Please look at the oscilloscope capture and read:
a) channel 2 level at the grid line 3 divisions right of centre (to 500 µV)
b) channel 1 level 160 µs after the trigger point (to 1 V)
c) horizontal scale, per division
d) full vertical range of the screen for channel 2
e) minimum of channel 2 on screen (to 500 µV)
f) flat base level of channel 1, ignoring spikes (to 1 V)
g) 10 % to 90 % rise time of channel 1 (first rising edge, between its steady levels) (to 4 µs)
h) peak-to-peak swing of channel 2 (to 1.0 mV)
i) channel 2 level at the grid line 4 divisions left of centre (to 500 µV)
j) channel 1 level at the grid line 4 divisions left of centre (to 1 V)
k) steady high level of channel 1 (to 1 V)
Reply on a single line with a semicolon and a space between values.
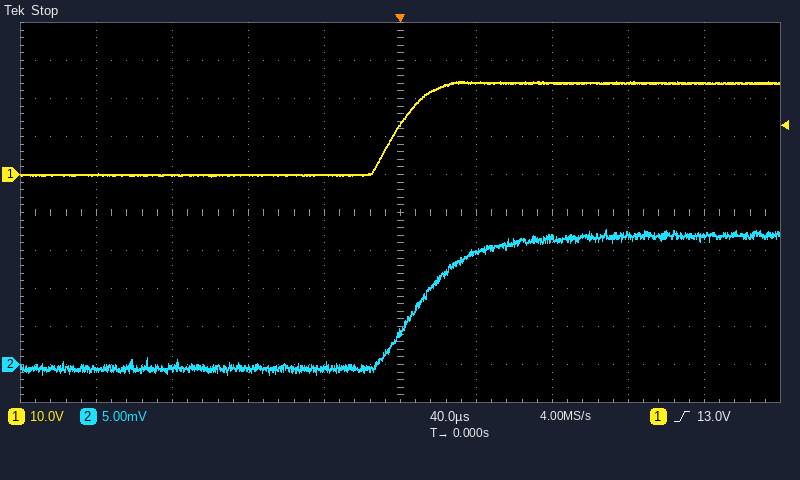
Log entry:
17.0 mV; 24 V; 40 µs; 50 mV; -1.5 mV; 0 V; 28 µs; 19.0 mV; -500 µV; 0 V; 24 V
